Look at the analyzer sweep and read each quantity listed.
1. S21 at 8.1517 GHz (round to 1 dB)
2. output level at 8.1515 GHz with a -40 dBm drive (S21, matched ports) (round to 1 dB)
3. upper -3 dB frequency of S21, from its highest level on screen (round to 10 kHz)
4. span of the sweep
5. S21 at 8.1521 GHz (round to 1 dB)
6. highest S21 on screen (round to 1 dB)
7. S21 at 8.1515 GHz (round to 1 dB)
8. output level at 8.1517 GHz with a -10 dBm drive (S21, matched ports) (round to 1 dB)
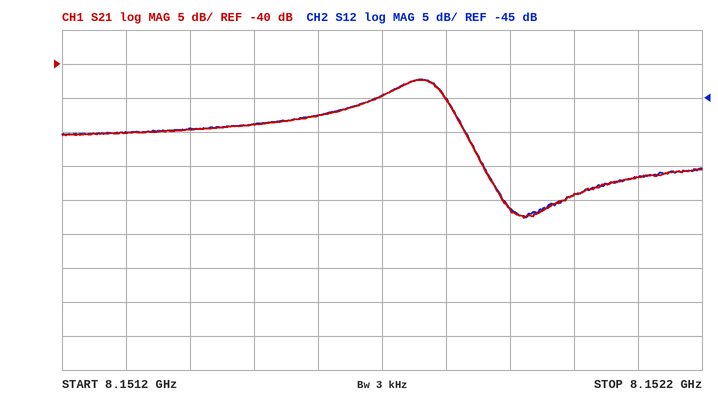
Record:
-45 dB
-89 dBm
8.15180 GHz
1 MHz
-57 dB
-42 dB
-49 dB
-55 dBm
